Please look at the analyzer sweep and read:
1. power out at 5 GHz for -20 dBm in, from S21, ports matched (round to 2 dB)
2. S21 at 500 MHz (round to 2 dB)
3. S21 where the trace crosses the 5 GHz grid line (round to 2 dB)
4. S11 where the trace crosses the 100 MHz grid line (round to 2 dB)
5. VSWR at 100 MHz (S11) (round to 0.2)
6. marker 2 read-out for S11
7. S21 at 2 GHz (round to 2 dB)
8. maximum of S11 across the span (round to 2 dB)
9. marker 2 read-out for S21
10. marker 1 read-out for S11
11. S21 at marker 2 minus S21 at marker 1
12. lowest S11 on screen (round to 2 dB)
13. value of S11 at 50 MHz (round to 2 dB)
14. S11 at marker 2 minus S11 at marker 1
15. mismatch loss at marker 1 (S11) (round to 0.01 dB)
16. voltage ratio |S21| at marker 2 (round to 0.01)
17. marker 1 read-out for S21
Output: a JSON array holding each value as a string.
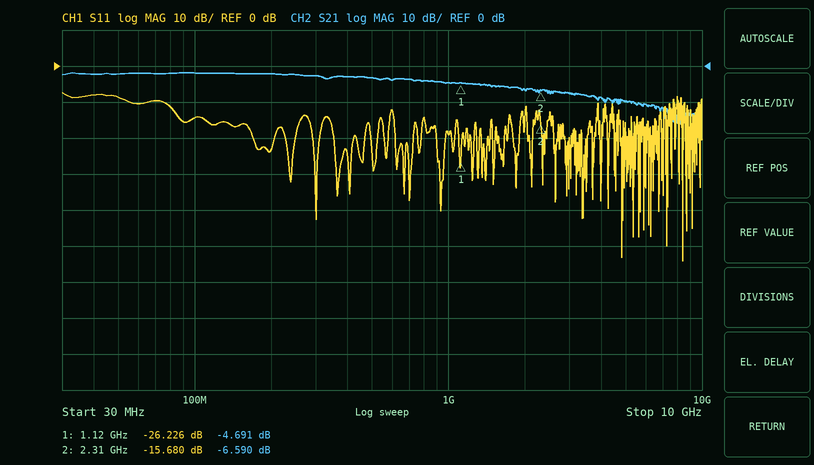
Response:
["-30 dBm", "-4 dB", "-10 dB", "-14 dB", "1.4", "-15.680 dB", "-6 dB", "-8 dB", "-6.590 dB", "-26.226 dB", "-1.899 dB", "-54 dB", "-8 dB", "10.546 dB", "0.01 dB", "0.47", "-4.691 dB"]
